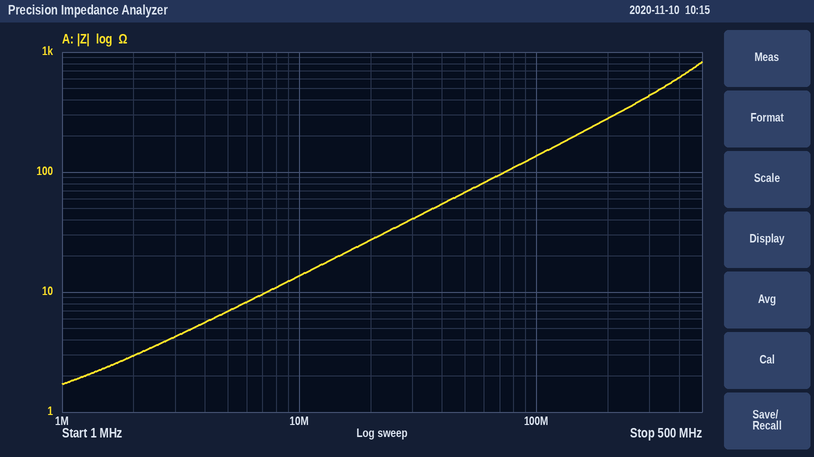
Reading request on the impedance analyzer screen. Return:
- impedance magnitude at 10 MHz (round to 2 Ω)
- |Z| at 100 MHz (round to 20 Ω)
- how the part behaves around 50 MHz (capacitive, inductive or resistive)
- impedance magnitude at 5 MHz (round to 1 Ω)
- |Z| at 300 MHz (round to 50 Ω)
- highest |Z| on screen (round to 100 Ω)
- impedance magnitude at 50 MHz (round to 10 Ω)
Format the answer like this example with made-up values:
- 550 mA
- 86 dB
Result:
- 14 Ω
- 140 Ω
- inductive
- 7 Ω
- 450 Ω
- 800 Ω
- 70 Ω
